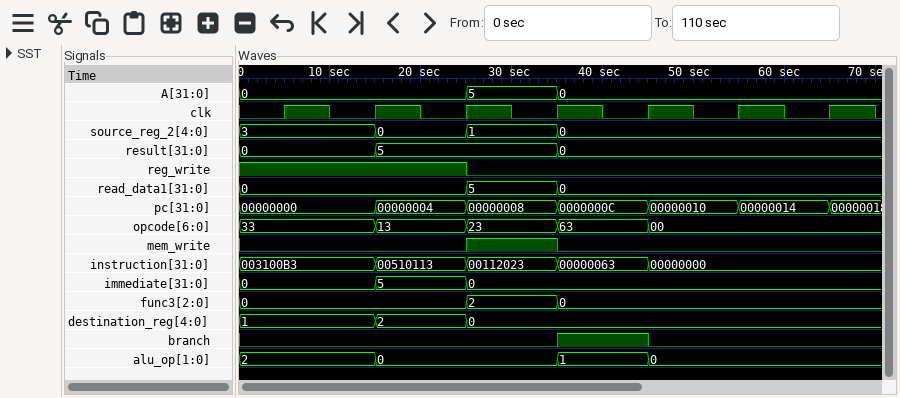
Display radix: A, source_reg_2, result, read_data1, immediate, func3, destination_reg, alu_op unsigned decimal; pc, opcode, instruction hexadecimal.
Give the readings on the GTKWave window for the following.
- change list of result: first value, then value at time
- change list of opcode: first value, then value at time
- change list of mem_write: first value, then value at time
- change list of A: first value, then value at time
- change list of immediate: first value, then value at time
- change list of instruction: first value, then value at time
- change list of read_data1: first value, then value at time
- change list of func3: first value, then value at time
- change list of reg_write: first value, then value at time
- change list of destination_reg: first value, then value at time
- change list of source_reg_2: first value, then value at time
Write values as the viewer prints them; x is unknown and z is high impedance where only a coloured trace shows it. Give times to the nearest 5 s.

0, 5 at 15 s, 0 at 35 s
33, 13 at 15 s, 23 at 25 s, 63 at 35 s, 00 at 45 s
0, 1 at 25 s, 0 at 35 s
0, 5 at 25 s, 0 at 35 s
0, 5 at 15 s, 0 at 25 s
003100B3, 00510113 at 15 s, 00112023 at 25 s, 00000063 at 35 s, 00000000 at 45 s
0, 5 at 25 s, 0 at 35 s
0, 2 at 25 s, 0 at 35 s
1, 0 at 25 s
1, 2 at 15 s, 0 at 25 s
3, 0 at 15 s, 1 at 25 s, 0 at 35 s
